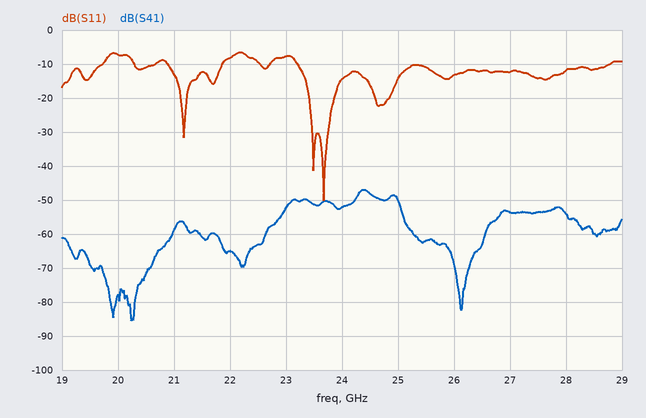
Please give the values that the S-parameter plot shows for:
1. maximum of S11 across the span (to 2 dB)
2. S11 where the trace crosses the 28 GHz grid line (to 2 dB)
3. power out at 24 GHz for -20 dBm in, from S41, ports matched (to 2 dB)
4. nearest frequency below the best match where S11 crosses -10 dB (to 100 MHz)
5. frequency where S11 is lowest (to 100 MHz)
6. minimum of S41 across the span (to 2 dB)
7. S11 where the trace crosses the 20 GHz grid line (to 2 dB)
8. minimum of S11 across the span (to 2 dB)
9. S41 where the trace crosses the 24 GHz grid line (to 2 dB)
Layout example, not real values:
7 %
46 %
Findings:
-6 dB
-12 dB
-72 dBm
23.2 GHz
23.7 GHz
-86 dB
-8 dB
-50 dB
-52 dB
